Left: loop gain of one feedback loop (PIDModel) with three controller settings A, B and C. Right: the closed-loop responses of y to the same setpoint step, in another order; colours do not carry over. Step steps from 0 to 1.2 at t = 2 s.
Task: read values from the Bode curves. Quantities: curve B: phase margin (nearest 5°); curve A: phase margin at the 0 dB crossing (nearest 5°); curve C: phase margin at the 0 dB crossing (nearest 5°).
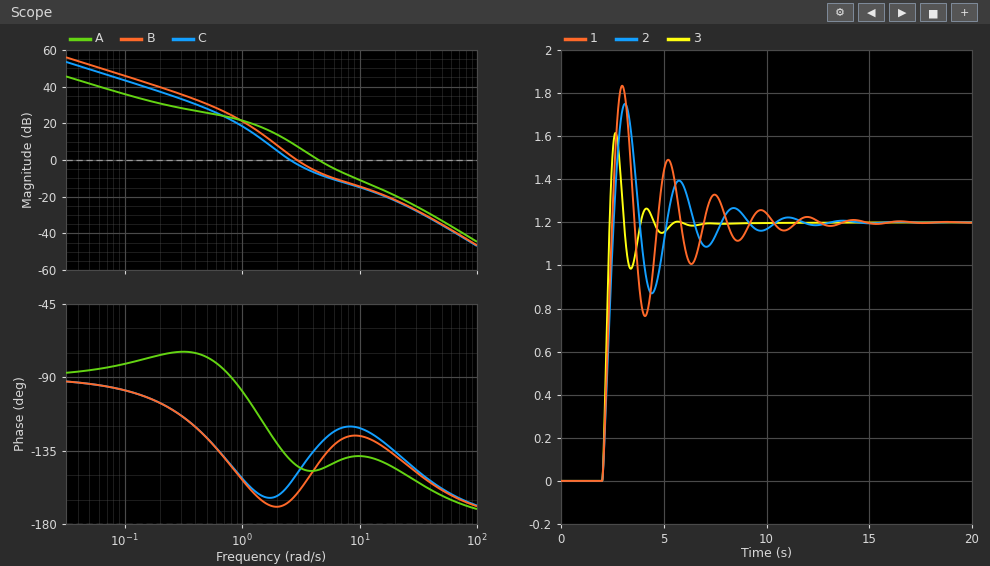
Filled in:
20°
35°
25°
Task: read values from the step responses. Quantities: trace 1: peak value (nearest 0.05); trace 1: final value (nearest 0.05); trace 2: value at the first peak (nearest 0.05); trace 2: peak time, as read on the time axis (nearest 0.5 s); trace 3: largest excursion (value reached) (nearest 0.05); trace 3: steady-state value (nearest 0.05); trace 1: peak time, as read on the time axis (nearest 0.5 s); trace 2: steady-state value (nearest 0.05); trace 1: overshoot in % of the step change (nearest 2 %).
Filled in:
1.85
1.20
1.75
3.0 s
1.60
1.20
3.0 s
1.20
52 %
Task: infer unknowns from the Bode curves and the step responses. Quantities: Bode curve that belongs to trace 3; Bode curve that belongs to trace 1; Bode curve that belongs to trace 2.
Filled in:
A
B
C
